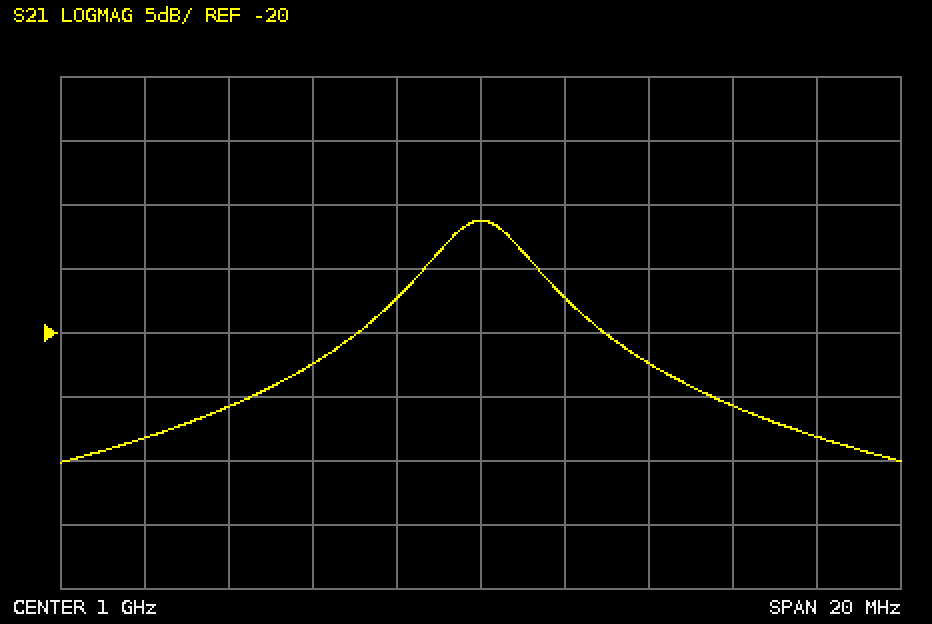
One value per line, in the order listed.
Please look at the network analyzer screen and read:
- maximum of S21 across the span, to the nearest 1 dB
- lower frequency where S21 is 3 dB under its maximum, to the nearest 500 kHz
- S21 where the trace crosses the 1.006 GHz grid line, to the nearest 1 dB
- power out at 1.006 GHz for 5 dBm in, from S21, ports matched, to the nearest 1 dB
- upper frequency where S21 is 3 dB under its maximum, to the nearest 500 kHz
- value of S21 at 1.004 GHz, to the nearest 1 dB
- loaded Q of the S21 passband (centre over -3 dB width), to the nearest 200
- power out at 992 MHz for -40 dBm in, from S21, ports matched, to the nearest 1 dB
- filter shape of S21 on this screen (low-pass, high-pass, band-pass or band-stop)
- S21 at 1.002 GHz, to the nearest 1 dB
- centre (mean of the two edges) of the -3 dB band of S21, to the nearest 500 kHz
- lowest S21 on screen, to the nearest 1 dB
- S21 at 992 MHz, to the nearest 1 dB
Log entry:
-11 dB
999.0 MHz
-26 dB
-21 dBm
1.0010 GHz
-22 dB
400
-68 dBm
band-pass
-17 dB
1.0000 GHz
-30 dB
-28 dB
